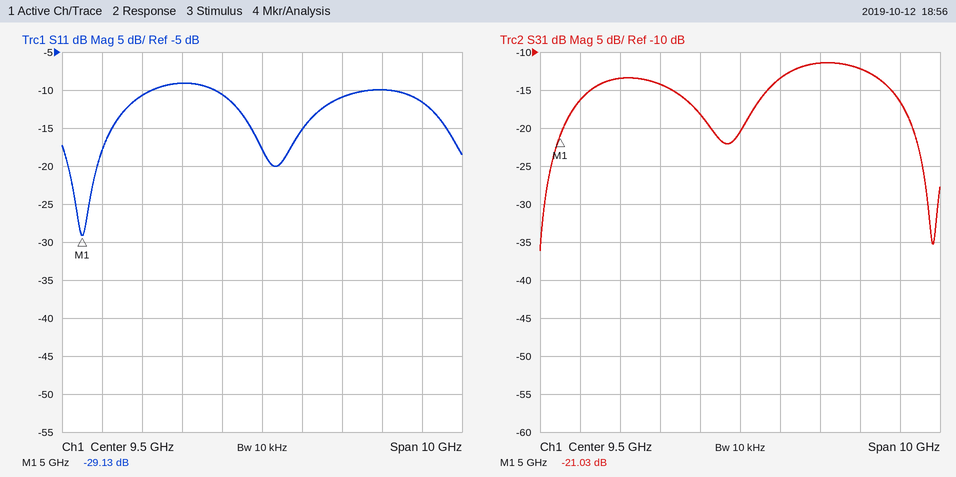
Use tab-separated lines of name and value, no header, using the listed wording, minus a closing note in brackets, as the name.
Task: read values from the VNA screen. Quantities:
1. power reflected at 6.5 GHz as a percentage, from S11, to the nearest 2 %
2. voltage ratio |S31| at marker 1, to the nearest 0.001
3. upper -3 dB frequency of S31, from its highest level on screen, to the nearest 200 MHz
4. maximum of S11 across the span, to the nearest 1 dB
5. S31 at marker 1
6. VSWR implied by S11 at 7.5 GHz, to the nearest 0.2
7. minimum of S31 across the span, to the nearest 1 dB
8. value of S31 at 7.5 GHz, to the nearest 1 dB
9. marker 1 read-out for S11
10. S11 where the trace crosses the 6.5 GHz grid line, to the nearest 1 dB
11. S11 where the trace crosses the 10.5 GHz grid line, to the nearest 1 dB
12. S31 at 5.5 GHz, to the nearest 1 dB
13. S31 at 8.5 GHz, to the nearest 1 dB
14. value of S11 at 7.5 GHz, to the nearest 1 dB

power reflected at 6.5 GHz as a percentage, from S11, to the nearest 2 %	8 %
voltage ratio |S31| at marker 1, to the nearest 0.001	0.089
upper -3 dB frequency of S31, from its highest level on screen, to the nearest 200 MHz	13.2 GHz
maximum of S11 across the span, to the nearest 1 dB	-9 dB
S31 at marker 1	-21.03 dB
VSWR implied by S11 at 7.5 GHz, to the nearest 0.2	2.0
minimum of S31 across the span, to the nearest 1 dB	-36 dB
value of S31 at 7.5 GHz, to the nearest 1 dB	-14 dB
marker 1 read-out for S11	-29.13 dB
S11 where the trace crosses the 6.5 GHz grid line, to the nearest 1 dB	-11 dB
S11 where the trace crosses the 10.5 GHz grid line, to the nearest 1 dB	-15 dB
S31 at 5.5 GHz, to the nearest 1 dB	-16 dB
S31 at 8.5 GHz, to the nearest 1 dB	-18 dB
value of S11 at 7.5 GHz, to the nearest 1 dB	-9 dB
